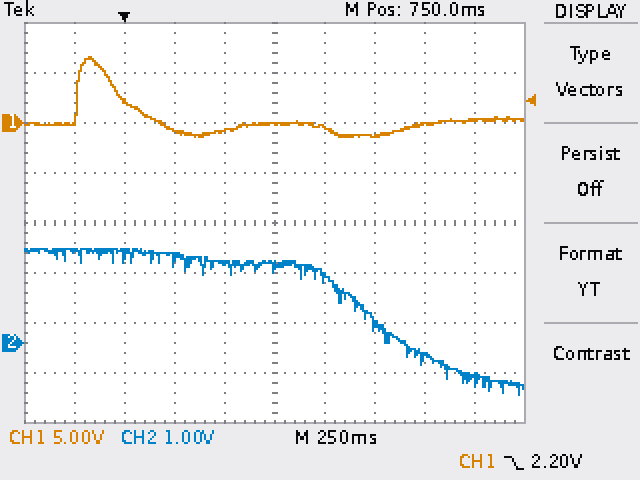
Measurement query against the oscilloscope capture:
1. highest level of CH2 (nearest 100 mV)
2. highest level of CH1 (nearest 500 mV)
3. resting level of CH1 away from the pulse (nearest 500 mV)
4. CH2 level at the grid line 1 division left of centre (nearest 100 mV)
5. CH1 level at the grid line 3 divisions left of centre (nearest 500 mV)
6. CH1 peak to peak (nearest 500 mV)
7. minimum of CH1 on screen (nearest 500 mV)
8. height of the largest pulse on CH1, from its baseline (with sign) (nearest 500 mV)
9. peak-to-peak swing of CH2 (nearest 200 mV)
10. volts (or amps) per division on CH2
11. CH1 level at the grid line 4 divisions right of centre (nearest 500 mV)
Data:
1.9 V
6.5 V
0.0 V
1.6 V
2.0 V
8.0 V
-1.5 V
+6.5 V
3.0 V
1 V
500 mV
